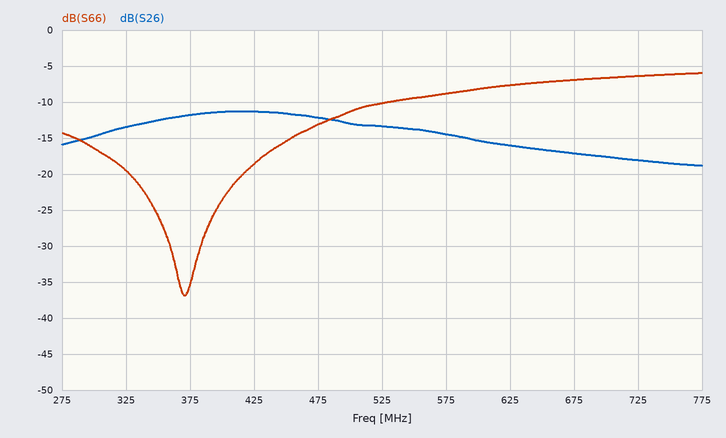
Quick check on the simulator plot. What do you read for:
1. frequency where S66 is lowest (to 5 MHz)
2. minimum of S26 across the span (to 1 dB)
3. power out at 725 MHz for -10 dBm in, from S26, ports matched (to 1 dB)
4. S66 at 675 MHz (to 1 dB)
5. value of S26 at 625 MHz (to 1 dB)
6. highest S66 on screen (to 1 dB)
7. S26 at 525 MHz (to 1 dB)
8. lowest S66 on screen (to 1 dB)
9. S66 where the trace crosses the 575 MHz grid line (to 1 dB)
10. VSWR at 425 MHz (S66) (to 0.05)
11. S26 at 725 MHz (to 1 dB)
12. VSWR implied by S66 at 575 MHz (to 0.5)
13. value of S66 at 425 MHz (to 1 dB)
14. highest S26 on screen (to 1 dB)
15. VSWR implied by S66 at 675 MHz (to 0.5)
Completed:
370 MHz
-19 dB
-28 dBm
-7 dB
-16 dB
-6 dB
-13 dB
-37 dB
-9 dB
1.25
-18 dB
2.0
-19 dB
-11 dB
2.5
